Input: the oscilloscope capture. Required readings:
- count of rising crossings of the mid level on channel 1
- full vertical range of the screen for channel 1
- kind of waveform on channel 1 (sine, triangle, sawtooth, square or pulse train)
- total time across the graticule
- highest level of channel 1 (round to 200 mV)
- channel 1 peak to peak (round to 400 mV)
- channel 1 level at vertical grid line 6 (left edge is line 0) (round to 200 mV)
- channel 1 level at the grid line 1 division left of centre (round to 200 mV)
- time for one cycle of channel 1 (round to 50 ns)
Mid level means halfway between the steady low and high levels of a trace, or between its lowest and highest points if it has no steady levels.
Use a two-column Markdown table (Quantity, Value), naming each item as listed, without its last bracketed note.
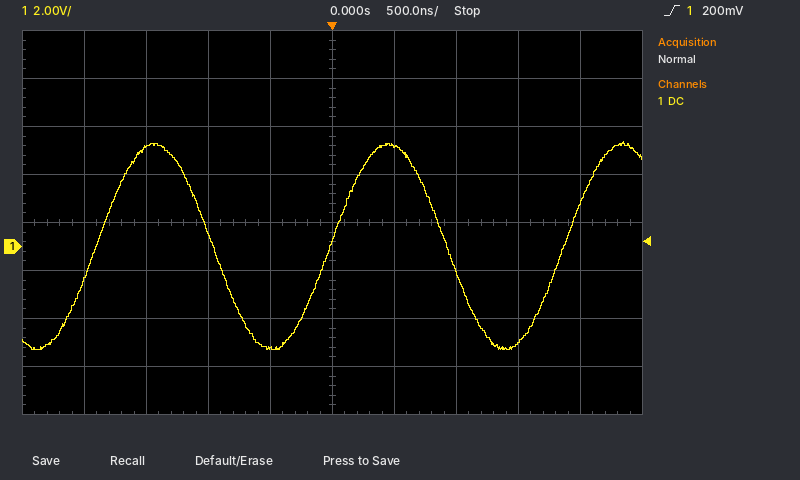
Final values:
| Quantity | Value |
|---|---|
| count of rising crossings of the mid level on channel 1 | 3 |
| full vertical range of the screen for channel 1 | 16 V |
| kind of waveform on channel 1 | sine |
| total time across the graticule | 5 µs |
| highest level of channel 1 | 4.4 V |
| channel 1 peak to peak | 8.8 V |
| channel 1 level at vertical grid line 6 (left edge is line 0) | 4.2 V |
| channel 1 level at the grid line 1 division left of centre | -4.2 V |
| time for one cycle of channel 1 | 1.90 µs |
